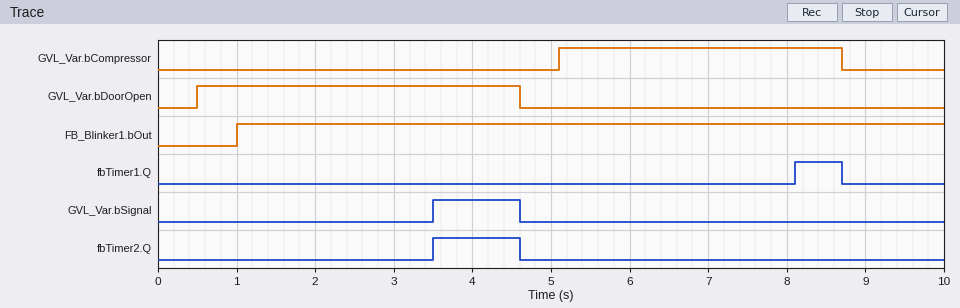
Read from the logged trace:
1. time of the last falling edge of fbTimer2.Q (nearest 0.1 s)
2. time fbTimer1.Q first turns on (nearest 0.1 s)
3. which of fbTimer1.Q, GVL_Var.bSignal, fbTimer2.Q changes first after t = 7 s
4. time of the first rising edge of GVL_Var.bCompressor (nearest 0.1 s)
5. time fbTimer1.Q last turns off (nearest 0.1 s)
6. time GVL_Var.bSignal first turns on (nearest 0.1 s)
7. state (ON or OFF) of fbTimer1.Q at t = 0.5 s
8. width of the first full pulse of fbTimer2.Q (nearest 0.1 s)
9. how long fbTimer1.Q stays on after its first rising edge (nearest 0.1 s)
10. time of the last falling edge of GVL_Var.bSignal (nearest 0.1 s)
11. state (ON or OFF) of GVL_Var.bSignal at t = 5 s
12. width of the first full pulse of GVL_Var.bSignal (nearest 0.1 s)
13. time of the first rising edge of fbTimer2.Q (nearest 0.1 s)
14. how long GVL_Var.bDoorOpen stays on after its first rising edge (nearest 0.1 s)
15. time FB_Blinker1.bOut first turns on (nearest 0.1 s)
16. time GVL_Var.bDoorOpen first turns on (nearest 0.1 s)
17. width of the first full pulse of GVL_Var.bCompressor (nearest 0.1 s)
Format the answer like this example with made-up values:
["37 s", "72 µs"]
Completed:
["4.6 s", "8.1 s", "fbTimer1.Q", "5.1 s", "8.7 s", "3.5 s", "OFF", "1.1 s", "0.6 s", "4.6 s", "OFF", "1.1 s", "3.5 s", "4.1 s", "1.0 s", "0.5 s", "3.6 s"]
